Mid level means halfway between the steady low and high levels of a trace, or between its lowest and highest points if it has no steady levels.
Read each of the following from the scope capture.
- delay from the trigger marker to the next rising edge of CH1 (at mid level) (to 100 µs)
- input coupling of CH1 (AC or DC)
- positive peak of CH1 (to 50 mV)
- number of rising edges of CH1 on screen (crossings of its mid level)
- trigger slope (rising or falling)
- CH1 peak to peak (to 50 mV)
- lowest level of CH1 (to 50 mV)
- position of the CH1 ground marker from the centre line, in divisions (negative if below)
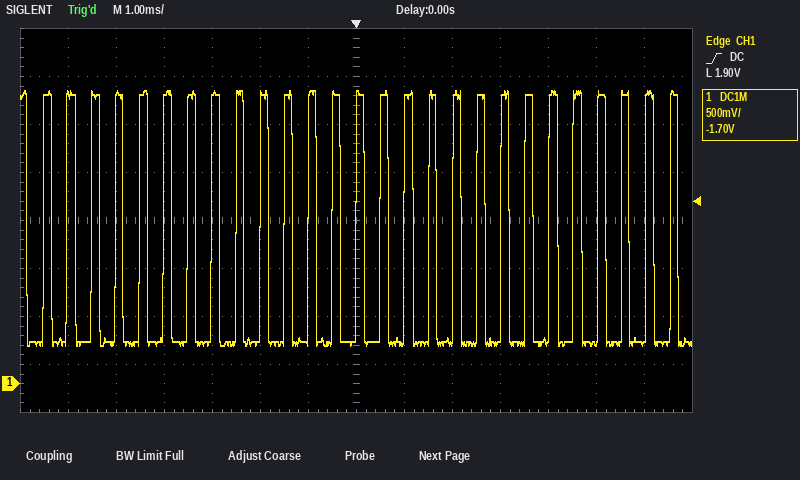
500 µs
DC
3.05 V
27
rising
2.65 V
400 mV
-3.4 div
